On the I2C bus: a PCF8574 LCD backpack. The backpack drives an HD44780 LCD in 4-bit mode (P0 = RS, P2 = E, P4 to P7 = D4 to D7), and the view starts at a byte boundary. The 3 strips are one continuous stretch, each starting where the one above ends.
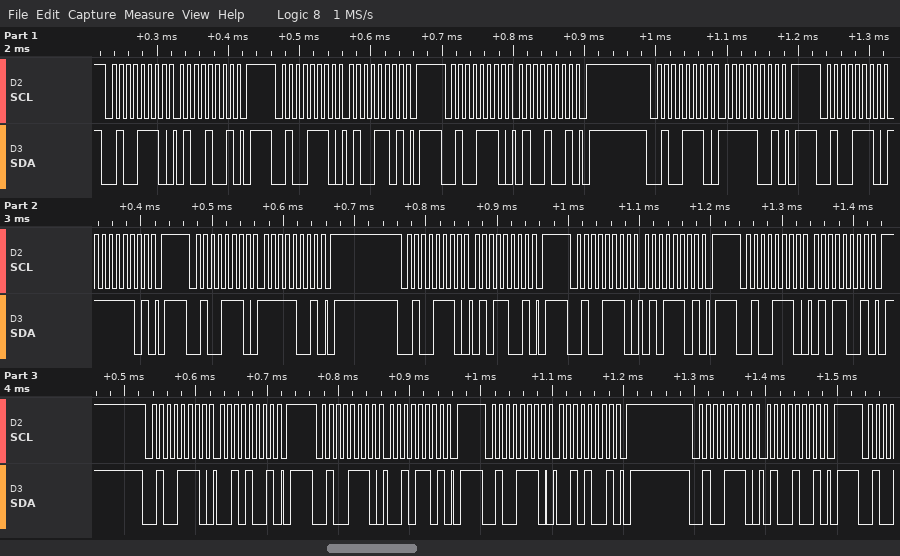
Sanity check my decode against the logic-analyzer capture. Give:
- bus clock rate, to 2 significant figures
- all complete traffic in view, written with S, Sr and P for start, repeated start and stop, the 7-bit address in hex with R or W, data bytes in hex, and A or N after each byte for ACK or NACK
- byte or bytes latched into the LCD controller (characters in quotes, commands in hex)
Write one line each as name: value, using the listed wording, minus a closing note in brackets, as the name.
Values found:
bus clock rate, to 2 significant figures: 100 kHz
all complete traffic in view, written with S, Sr and P for start, repeated start and stop, the 7-bit address in hex with R or W, data bytes in hex, and A or N after each byte for ACK or NACK: S 27W A 49 A P S 27W A 4D A P S 27W A 49 A P S 27W A F9 A P S 27W A FD A P S 27W A F9 A P S 27W A 59 A P S 27W A 5D A P S 27W A 59 A P S 27W A 29 A P S 27W A 2D A P S 27W A 29 A P S 27W A 49 A P
byte or bytes latched into the LCD controller: 'O' 'R'
